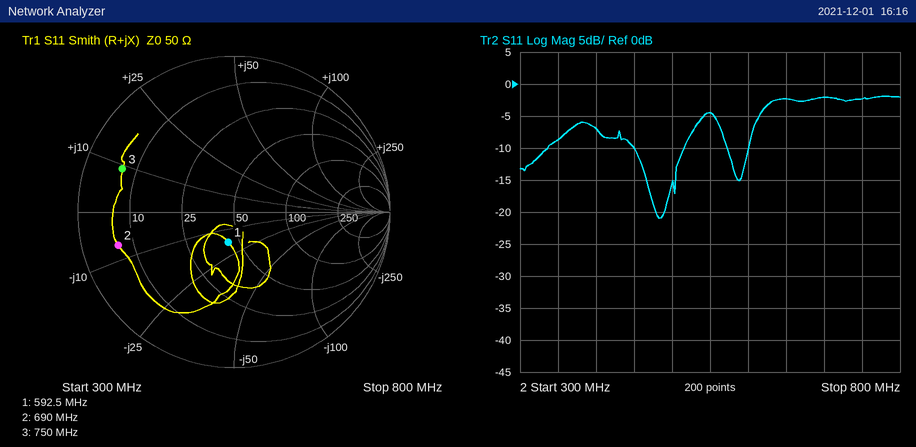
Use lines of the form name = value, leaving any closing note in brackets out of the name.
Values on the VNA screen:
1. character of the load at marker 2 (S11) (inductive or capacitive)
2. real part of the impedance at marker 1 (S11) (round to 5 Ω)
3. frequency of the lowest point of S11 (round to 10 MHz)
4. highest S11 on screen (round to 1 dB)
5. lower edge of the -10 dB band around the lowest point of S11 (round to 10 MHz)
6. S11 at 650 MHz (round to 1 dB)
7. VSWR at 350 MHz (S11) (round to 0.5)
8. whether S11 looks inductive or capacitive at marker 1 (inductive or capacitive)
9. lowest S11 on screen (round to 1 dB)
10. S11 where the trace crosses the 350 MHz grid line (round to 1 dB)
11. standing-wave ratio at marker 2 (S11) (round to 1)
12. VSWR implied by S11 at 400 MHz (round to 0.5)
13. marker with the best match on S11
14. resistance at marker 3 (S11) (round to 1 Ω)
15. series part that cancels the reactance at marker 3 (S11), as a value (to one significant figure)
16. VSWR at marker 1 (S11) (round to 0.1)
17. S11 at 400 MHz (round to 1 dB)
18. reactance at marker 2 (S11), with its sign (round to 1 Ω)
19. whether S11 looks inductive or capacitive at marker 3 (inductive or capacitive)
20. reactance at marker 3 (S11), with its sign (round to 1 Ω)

character of the load at marker 2 (S11) = capacitive
real part of the impedance at marker 1 (S11) = 45 Ω
frequency of the lowest point of S11 = 480 MHz
highest S11 on screen = -2 dB
lower edge of the -10 dB band around the lowest point of S11 = 450 MHz
S11 at 650 MHz = -2 dB
VSWR at 350 MHz (S11) = 2.0
whether S11 looks inductive or capacitive at marker 1 = capacitive
lowest S11 on screen = -21 dB
S11 where the trace crosses the 350 MHz grid line = -9 dB
standing-wave ratio at marker 2 (S11) = 8
VSWR implied by S11 at 400 MHz = 2.5
marker with the best match on S11 = marker 1
resistance at marker 3 (S11) = 7 Ω
series part that cancels the reactance at marker 3 (S11), as a value = 20 pF
VSWR at marker 1 (S11) = 1.5
S11 at 400 MHz = -7 dB
reactance at marker 2 (S11), with its sign = -7 Ω
whether S11 looks inductive or capacitive at marker 3 = inductive
reactance at marker 3 (S11), with its sign = +9 Ω
